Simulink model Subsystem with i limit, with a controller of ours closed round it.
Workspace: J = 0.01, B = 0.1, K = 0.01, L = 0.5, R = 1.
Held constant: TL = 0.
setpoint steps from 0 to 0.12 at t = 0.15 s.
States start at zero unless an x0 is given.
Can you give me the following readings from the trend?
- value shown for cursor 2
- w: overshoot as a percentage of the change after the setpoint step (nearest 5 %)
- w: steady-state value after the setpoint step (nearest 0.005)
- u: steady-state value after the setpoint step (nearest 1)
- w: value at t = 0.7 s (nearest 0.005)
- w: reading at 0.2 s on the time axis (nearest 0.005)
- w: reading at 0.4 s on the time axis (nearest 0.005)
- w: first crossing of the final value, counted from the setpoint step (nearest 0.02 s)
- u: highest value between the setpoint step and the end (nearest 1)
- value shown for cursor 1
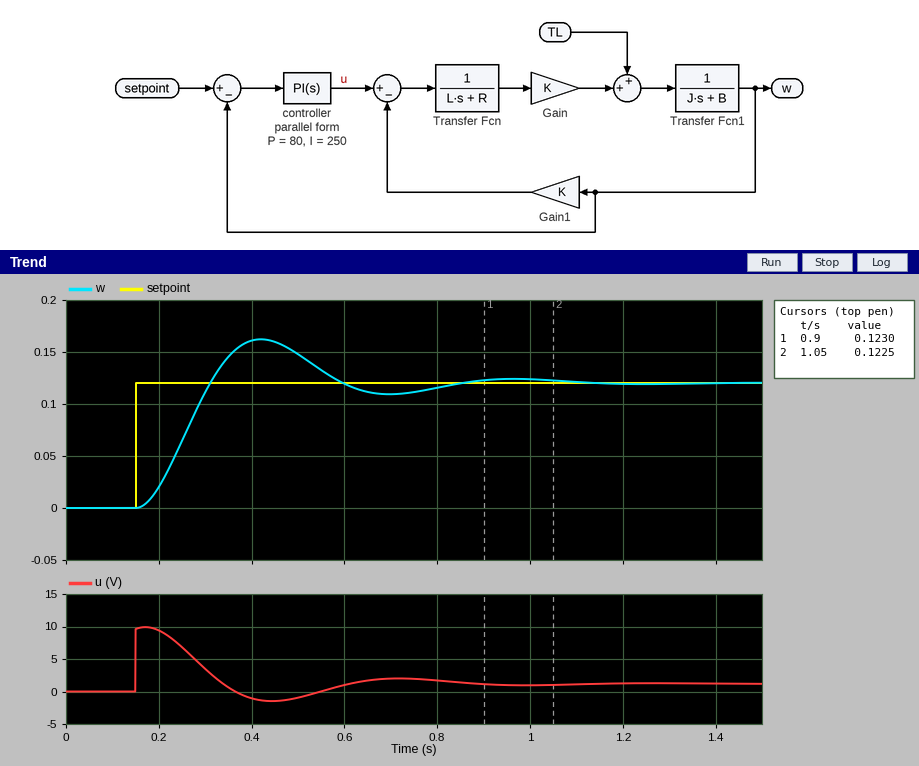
0.1225
35 %
0.120
1
0.110
0.020
0.160
0.16 s
10
0.1230
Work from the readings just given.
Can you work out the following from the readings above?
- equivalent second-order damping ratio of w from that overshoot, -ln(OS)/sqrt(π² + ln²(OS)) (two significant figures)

0.32
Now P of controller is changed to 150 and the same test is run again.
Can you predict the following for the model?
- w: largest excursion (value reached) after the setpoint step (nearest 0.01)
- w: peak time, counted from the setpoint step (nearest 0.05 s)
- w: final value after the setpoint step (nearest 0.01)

0.16
0.20 s
0.12
